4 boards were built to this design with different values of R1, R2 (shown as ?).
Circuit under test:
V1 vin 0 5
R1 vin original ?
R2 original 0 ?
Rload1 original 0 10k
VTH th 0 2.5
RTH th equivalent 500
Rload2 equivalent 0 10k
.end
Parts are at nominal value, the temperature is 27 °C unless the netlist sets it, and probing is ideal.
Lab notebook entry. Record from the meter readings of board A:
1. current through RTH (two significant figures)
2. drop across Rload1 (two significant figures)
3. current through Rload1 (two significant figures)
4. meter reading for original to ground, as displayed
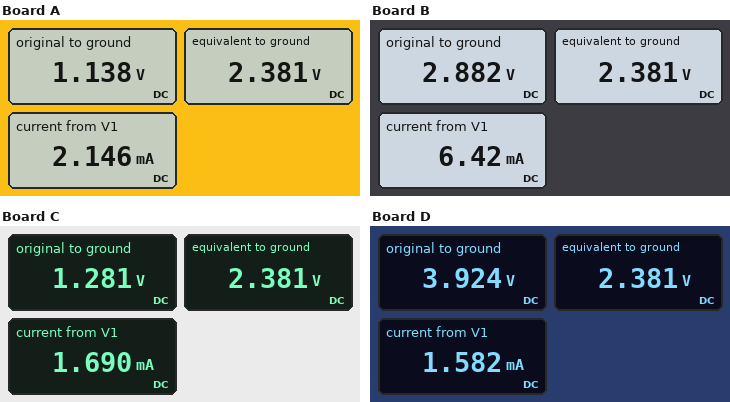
240 µA
1.1 V
110 µA
1.138 V
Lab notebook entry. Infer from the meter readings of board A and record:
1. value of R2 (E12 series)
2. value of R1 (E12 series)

560 Ω
1.8 kΩ
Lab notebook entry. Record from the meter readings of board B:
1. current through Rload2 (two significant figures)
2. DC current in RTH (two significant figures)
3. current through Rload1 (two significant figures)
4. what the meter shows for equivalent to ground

240 µA
240 µA
290 µA
2.381 V
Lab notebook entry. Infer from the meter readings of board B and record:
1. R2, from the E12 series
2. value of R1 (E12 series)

470 Ω
330 Ω
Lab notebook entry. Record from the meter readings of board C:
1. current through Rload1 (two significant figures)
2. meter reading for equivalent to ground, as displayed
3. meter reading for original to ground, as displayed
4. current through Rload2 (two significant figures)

130 µA
2.381 V
1.281 V
240 µA
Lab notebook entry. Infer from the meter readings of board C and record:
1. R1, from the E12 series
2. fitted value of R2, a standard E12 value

2.2 kΩ
820 Ω
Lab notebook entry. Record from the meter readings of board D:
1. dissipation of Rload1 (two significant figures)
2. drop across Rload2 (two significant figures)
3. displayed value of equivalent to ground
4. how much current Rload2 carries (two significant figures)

1.5 mW
2.4 V
2.381 V
240 µA
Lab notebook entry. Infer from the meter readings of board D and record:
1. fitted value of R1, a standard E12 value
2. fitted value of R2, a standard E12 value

680 Ω
3.3 kΩ
